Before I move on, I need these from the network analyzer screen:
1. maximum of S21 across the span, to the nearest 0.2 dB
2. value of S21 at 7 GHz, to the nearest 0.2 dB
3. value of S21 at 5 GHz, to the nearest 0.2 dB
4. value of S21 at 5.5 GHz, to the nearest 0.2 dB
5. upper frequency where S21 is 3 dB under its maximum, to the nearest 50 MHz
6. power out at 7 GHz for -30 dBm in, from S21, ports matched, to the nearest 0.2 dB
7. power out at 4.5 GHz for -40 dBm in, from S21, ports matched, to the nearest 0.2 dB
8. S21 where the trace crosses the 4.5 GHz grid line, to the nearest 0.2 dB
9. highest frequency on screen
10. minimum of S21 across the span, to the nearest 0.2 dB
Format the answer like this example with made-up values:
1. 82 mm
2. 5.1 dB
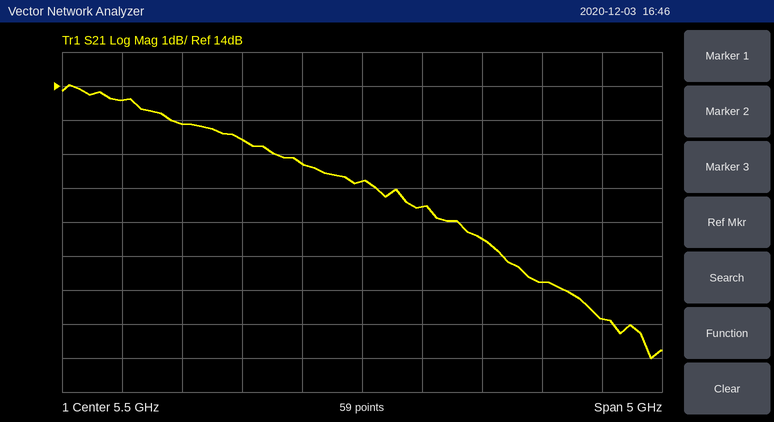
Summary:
1. 14.0 dB
2. 8.2 dB
3. 11.8 dB
4. 11.2 dB
5. 5.60 GHz
6. -21.8 dBm
7. -27.6 dBm
8. 12.4 dB
9. 8 GHz
10. 6.0 dB
